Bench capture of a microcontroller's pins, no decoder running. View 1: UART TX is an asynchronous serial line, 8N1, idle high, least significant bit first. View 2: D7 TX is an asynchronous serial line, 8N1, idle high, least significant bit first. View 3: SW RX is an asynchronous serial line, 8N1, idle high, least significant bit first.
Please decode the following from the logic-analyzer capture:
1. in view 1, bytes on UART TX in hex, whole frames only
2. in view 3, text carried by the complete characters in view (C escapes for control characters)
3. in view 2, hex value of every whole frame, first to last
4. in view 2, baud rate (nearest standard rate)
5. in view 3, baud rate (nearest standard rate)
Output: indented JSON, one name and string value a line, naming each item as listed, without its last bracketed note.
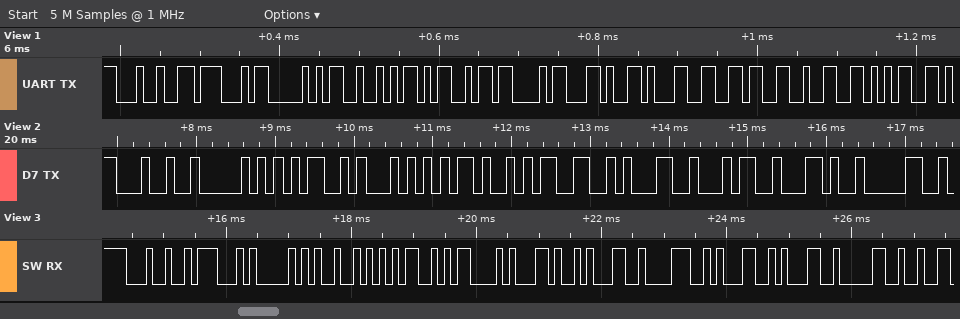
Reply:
{
  "in view 1, bytes on UART TX in hex, whole frames only": "24 47 50 52 4D 43 2C 31 36 32 35",
  "in view 3, text carried by the complete characters in view": "\"$GPRMC,18110\"",
  "in view 2, hex value of every whole frame, first to last": "24 50 4D 54 4B 33 31 34 2C 30",
  "in view 2, baud rate": "9600 baud",
  "in view 3, baud rate": "9600 baud"
}
